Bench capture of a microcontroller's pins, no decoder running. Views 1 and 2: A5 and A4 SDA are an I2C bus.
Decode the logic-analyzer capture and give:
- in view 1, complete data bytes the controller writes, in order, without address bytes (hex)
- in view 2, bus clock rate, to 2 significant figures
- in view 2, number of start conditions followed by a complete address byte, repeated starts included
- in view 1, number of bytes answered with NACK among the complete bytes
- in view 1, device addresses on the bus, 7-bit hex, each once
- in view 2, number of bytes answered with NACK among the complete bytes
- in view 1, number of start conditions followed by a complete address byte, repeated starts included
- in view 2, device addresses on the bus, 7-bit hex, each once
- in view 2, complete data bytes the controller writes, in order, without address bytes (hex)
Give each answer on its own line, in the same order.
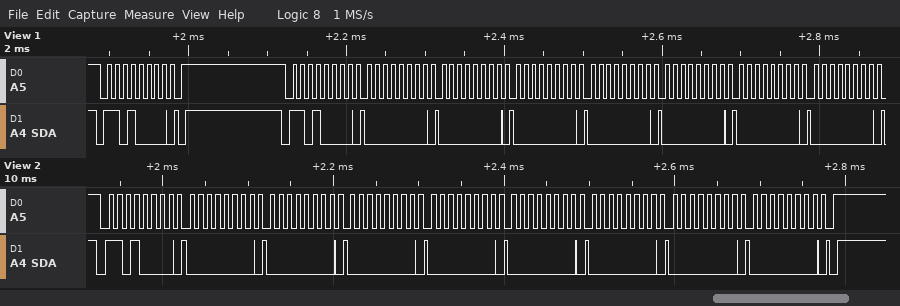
00 00 00 00 00 00 00
100 kHz
1
0
0x68
0
2
0x68
00 00 00 00 00 00 00 00
